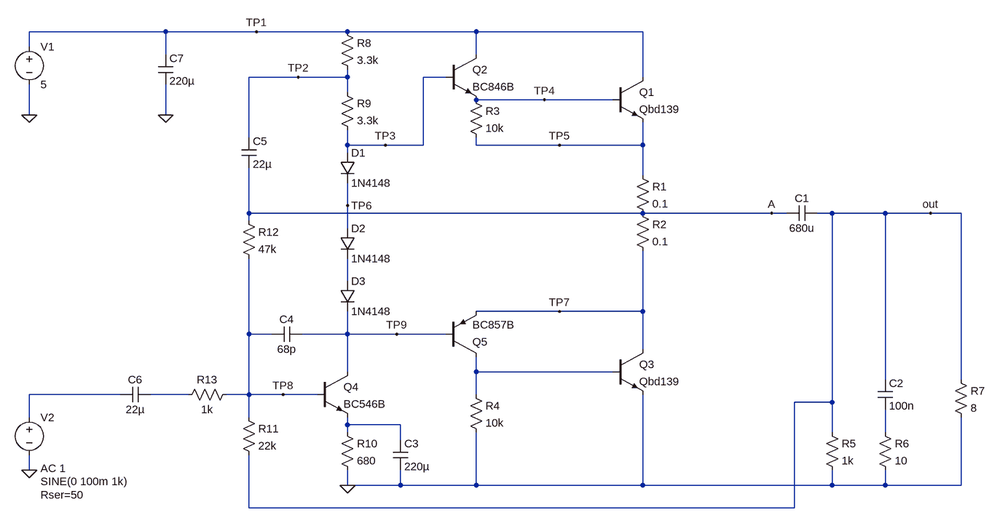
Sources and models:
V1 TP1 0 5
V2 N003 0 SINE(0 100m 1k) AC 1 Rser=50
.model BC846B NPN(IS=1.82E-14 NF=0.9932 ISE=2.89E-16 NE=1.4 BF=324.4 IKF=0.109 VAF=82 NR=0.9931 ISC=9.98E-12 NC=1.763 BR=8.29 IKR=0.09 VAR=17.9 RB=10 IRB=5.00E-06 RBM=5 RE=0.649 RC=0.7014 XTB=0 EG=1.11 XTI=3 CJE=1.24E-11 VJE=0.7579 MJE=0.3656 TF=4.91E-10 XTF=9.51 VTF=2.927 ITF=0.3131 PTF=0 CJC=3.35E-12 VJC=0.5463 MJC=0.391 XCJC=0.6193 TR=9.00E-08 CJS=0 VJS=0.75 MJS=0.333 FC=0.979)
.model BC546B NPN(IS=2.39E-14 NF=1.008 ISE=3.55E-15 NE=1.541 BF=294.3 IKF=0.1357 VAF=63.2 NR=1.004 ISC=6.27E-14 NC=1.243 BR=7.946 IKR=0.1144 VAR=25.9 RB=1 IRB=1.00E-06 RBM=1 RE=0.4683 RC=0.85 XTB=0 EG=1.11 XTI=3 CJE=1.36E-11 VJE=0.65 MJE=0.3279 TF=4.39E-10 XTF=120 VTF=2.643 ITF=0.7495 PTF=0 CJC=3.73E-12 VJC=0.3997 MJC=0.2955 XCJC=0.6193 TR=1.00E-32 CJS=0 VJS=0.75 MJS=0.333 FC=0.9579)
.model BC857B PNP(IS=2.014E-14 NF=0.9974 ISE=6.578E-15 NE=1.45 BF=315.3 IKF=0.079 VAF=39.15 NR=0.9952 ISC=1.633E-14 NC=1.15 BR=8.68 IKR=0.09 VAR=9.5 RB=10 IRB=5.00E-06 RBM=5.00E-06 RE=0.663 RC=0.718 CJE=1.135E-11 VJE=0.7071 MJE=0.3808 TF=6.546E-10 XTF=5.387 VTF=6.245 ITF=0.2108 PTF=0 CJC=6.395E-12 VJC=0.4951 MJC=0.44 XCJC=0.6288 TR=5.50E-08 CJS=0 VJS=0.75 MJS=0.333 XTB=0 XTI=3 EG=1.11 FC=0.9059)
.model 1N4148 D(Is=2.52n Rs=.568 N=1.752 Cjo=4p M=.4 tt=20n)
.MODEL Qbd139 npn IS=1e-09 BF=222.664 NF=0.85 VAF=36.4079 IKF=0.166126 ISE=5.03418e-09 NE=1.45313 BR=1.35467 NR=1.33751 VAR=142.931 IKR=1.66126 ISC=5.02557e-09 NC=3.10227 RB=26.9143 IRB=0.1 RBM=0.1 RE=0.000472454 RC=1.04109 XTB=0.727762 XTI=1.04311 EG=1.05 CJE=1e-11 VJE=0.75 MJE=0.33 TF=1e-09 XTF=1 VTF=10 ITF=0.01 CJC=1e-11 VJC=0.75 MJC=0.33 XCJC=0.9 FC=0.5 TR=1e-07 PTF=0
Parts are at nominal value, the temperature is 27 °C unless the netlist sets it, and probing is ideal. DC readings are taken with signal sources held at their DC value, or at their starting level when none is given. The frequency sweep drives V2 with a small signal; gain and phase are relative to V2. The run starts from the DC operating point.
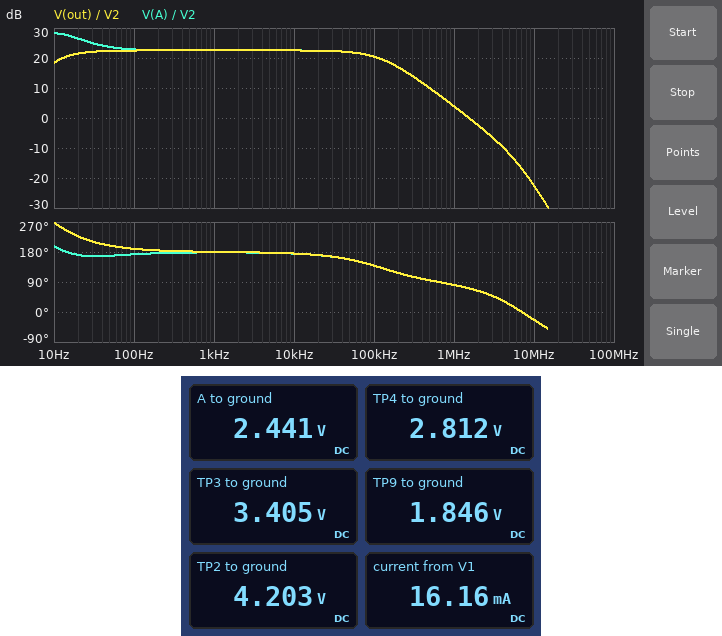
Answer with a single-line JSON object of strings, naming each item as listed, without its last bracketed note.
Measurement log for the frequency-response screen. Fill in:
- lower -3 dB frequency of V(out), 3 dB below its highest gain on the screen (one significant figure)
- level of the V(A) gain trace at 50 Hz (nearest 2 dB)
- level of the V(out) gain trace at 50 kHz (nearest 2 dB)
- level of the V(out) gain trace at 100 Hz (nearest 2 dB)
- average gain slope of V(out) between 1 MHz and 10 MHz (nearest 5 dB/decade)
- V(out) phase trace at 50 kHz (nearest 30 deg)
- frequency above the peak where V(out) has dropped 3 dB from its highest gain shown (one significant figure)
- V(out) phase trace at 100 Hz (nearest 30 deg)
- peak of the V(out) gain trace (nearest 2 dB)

{"lower -3 dB frequency of V(out), 3 dB below its highest gain on the screen": "10 Hz", "level of the V(A) gain trace at 50 Hz": "24 dB", "level of the V(out) gain trace at 50 kHz": "22 dB", "level of the V(out) gain trace at 100 Hz": "22 dB", "average gain slope of V(out) between 1 MHz and 10 MHz": "-25 dB/decade", "V(out) phase trace at 50 kHz": "150 deg", "frequency above the peak where V(out) has dropped 3 dB from its highest gain shown": "100 kHz", "V(out) phase trace at 100 Hz": "180 deg", "peak of the V(out) gain trace": "22 dB"}
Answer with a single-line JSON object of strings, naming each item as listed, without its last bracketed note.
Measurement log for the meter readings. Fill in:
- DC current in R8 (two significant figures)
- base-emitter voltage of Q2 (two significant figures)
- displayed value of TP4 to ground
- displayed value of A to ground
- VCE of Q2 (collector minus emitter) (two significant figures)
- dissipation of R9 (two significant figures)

{"DC current in R8": "240 µA", "base-emitter voltage of Q2": "590 mV", "displayed value of TP4 to ground": "2.812 V", "displayed value of A to ground": "2.441 V", "VCE of Q2 (collector minus emitter)": "2.2 V", "dissipation of R9": "190 µW"}
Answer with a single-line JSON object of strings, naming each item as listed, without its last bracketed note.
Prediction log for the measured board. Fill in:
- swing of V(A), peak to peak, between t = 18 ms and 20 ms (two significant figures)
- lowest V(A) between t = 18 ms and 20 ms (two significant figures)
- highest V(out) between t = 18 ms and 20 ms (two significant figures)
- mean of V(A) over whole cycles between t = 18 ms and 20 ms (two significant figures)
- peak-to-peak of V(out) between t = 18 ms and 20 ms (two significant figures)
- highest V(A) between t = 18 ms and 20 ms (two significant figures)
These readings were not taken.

{"swing of V(A), peak to peak, between t = 18 ms and 20 ms": "2.7 V", "lowest V(A) between t = 18 ms and 20 ms": "1.1 V", "highest V(out) between t = 18 ms and 20 ms": "1.3 V", "mean of V(A) over whole cycles between t = 18 ms and 20 ms": "2.4 V", "peak-to-peak of V(out) between t = 18 ms and 20 ms": "2.7 V", "highest V(A) between t = 18 ms and 20 ms": "3.7 V"}
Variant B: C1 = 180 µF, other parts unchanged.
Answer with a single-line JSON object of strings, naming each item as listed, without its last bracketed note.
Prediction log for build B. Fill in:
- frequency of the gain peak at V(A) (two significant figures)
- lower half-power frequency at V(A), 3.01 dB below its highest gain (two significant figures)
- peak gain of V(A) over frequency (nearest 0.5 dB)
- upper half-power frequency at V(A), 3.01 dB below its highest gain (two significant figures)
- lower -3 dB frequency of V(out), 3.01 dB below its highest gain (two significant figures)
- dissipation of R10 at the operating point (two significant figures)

{"frequency of the gain peak at V(A)": "18 Hz", "lower half-power frequency at V(A), 3.01 dB below its highest gain": "7.2 Hz", "peak gain of V(A) over frequency": "31.5 dB", "upper half-power frequency at V(A), 3.01 dB below its highest gain": "54 Hz", "lower -3 dB frequency of V(out), 3.01 dB below its highest gain": "34 Hz", "dissipation of R10 at the operating point": "40 µW"}
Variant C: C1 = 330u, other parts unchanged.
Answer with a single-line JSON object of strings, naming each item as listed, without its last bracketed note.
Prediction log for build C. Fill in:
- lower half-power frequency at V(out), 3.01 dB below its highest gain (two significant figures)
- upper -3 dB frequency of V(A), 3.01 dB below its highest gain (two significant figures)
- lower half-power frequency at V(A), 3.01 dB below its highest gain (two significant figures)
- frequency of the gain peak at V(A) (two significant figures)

{"lower half-power frequency at V(out), 3.01 dB below its highest gain": "20 Hz", "upper -3 dB frequency of V(A), 3.01 dB below its highest gain": "37 Hz", "lower half-power frequency at V(A), 3.01 dB below its highest gain": "6.2 Hz", "frequency of the gain peak at V(A)": "14 Hz"}
